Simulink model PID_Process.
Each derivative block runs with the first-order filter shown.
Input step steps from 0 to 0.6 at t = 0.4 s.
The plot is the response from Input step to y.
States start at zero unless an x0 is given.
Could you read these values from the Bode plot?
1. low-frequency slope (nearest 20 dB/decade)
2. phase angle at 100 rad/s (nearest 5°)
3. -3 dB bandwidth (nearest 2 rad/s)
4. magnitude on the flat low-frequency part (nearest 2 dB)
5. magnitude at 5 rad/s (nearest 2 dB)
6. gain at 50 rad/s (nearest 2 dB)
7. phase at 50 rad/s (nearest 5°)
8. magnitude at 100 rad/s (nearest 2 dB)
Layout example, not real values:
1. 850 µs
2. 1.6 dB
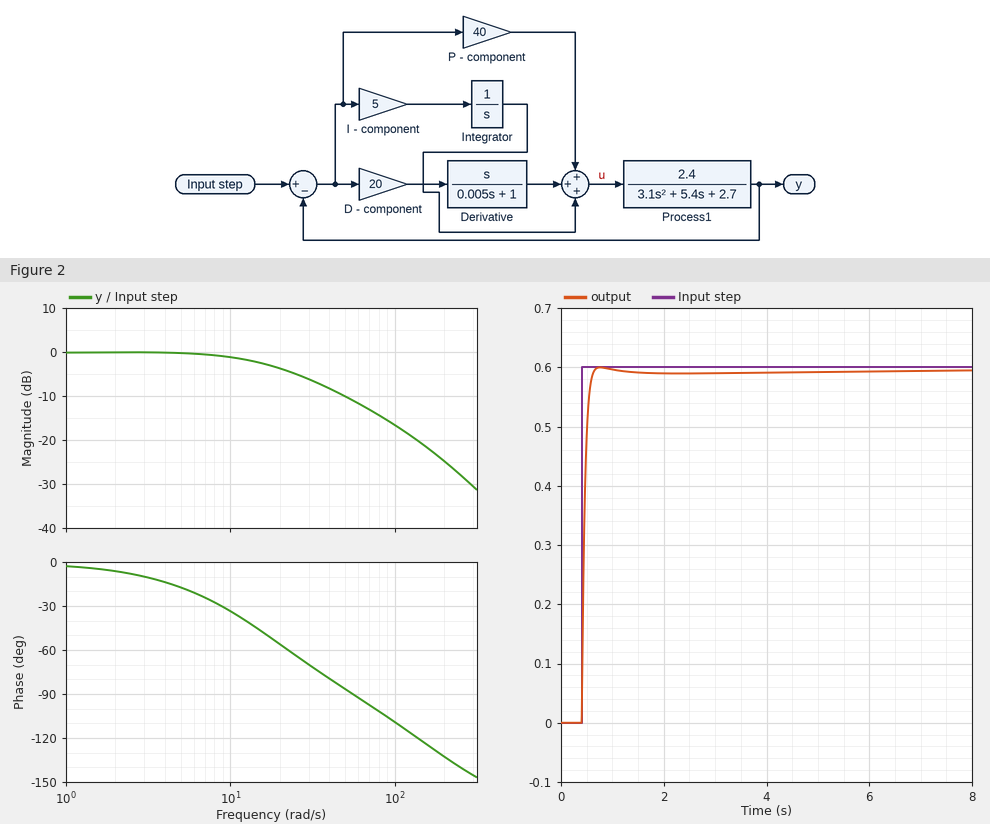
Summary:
1. 0 dB/decade
2. -110°
3. 18 rad/s
4. 0 dB
5. 0 dB
6. -10 dB
7. -85°
8. -16 dB
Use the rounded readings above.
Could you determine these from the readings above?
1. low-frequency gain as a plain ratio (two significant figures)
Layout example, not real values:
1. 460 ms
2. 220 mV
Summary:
1. 1.0
